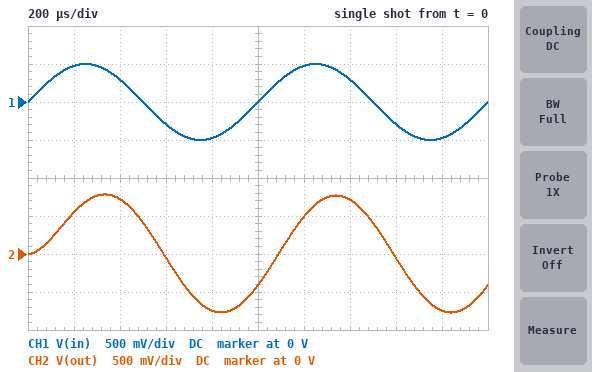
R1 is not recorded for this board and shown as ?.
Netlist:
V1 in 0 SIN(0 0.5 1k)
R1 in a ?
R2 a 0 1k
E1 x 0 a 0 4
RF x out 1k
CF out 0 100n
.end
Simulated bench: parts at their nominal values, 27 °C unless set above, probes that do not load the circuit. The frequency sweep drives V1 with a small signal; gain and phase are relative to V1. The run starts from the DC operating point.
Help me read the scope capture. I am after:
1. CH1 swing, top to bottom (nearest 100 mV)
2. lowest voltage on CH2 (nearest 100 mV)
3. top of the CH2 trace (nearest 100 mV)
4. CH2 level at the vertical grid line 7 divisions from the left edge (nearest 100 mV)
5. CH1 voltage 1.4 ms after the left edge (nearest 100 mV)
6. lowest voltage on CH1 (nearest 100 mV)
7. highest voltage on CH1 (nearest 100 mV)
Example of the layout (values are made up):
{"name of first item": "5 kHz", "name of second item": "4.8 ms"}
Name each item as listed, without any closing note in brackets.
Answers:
{"CH1 swing, top to bottom": "1.0 V", "lowest voltage on CH2": "-800 mV", "top of the CH2 trace": "800 mV", "CH2 level at the vertical grid line 7 divisions from the left edge": "700 mV", "CH1 voltage 1.4 ms after the left edge": "300 mV", "lowest voltage on CH1": "-500 mV", "highest voltage on CH1": "500 mV"}
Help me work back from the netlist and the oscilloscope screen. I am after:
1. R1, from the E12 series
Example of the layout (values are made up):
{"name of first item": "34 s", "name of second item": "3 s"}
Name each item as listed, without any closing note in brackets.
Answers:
{"R1, from the E12 series": "1.2 kΩ"}
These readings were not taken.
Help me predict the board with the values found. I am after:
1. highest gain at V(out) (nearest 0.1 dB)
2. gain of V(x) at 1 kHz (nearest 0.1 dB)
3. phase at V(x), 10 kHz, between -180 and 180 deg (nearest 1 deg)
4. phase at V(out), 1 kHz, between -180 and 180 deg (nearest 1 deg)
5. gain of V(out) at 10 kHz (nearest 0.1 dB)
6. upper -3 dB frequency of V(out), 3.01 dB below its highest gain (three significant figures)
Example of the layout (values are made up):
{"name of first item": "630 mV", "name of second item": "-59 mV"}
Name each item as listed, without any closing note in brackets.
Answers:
{"highest gain at V(out)": "5.2 dB", "gain of V(x) at 1 kHz": "5.2 dB", "phase at V(x), 10 kHz, between -180 and 180 deg": "0 deg", "phase at V(out), 1 kHz, between -180 and 180 deg": "-32 deg", "gain of V(out) at 10 kHz": "-10.9 dB", "upper -3 dB frequency of V(out), 3.01 dB below its highest gain": "1.59 kHz"}
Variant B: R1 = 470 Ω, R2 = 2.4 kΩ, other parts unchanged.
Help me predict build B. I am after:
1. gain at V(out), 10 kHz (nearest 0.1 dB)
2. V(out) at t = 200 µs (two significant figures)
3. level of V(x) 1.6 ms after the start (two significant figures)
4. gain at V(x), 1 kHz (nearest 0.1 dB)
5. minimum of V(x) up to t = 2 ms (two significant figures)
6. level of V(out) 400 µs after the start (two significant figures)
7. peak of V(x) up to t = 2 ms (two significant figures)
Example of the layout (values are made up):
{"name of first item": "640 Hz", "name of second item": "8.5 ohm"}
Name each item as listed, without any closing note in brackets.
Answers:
{"gain at V(out), 10 kHz": "-5.6 dB", "V(out) at t = 200 µs": "1.0 V", "level of V(x) 1.6 ms after the start": "-980 mV", "gain at V(x), 1 kHz": "10.5 dB", "minimum of V(x) up to t = 2 ms": "-1.7 V", "level of V(out) 400 µs after the start": "1.3 V", "peak of V(x) up to t = 2 ms": "1.7 V"}
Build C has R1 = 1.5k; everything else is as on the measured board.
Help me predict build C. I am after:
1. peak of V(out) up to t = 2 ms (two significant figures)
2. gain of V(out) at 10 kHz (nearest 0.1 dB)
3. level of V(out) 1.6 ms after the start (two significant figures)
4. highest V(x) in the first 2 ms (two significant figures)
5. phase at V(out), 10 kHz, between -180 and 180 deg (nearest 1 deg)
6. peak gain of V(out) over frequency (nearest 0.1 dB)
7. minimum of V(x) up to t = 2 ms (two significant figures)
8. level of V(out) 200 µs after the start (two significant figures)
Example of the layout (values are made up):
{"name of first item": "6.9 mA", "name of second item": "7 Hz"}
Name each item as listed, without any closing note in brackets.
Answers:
{"peak of V(out) up to t = 2 ms": "690 mV", "gain of V(out) at 10 kHz": "-12.0 dB", "level of V(out) 1.6 ms after the start": "-46 mV", "highest V(x) in the first 2 ms": "800 mV", "phase at V(out), 10 kHz, between -180 and 180 deg": "-81 deg", "peak gain of V(out) over frequency": "4.1 dB", "minimum of V(x) up to t = 2 ms": "-800 mV", "level of V(out) 200 µs after the start": "480 mV"}
